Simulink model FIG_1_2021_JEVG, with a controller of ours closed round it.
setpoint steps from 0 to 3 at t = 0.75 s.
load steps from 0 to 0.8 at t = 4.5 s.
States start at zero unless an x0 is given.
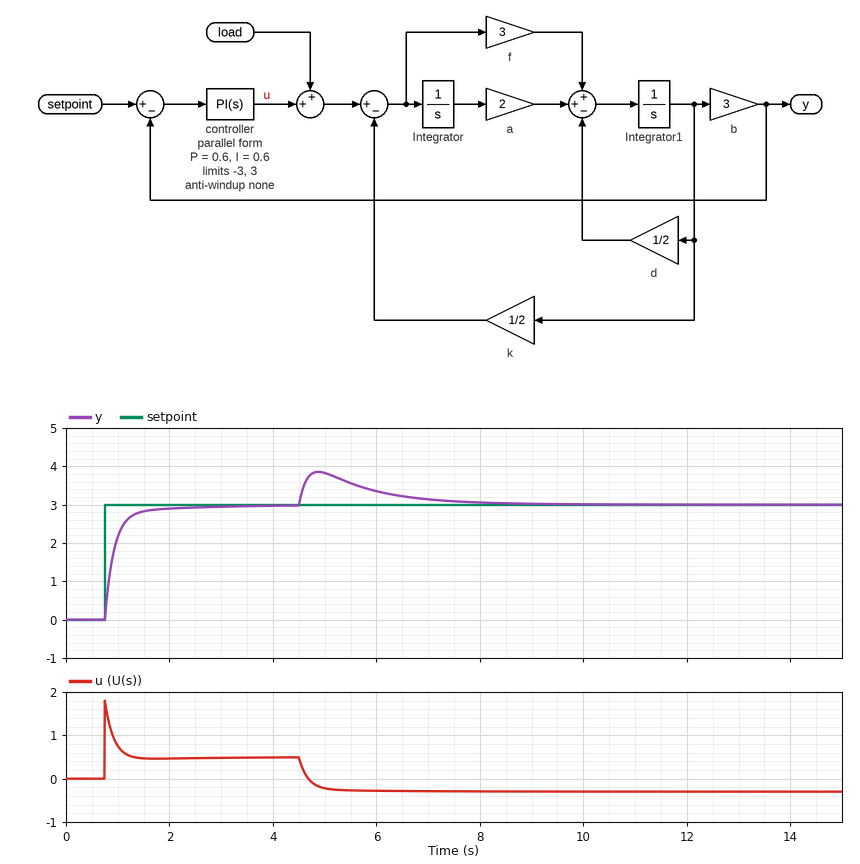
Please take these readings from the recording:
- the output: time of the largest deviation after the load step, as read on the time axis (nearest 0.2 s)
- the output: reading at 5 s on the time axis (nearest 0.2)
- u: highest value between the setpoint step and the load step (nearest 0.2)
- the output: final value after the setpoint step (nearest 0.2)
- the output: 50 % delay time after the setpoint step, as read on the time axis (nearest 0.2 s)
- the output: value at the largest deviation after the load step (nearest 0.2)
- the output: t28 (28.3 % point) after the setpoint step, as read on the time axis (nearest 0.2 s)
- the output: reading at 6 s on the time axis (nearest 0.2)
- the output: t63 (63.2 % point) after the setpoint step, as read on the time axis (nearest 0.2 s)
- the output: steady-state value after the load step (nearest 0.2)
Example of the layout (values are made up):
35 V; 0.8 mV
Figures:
4.8 s; 3.8; 1.8; 3.0; 0.8 s; 3.8; 0.8 s; 3.4; 1.0 s; 3.0
